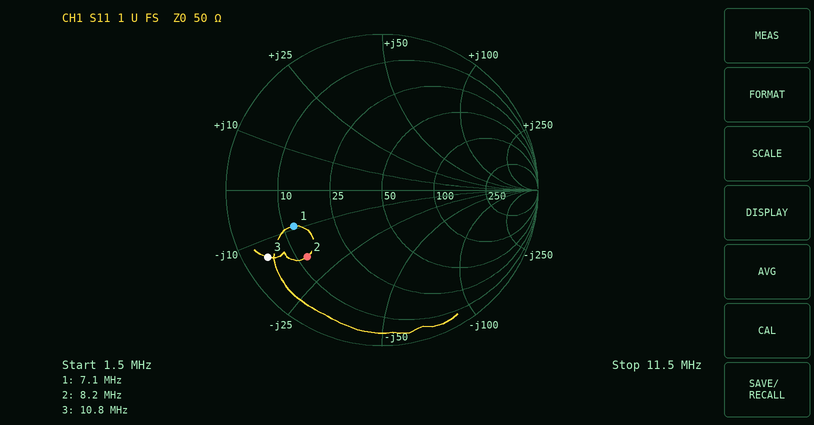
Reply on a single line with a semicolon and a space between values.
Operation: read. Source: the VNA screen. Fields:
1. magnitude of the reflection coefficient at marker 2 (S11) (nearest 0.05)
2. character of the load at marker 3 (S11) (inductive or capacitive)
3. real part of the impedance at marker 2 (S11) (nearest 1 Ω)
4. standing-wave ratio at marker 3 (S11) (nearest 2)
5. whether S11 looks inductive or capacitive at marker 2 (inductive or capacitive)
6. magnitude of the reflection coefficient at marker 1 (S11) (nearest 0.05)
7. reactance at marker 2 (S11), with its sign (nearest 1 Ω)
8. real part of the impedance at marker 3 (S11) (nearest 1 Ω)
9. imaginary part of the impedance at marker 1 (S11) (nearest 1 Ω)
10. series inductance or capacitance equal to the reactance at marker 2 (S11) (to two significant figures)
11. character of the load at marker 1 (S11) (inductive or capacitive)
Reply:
0.65; capacitive; 12 Ω; 12; capacitive; 0.60; -18 Ω; 4 Ω; -9 Ω; 1.1 nF; capacitive
